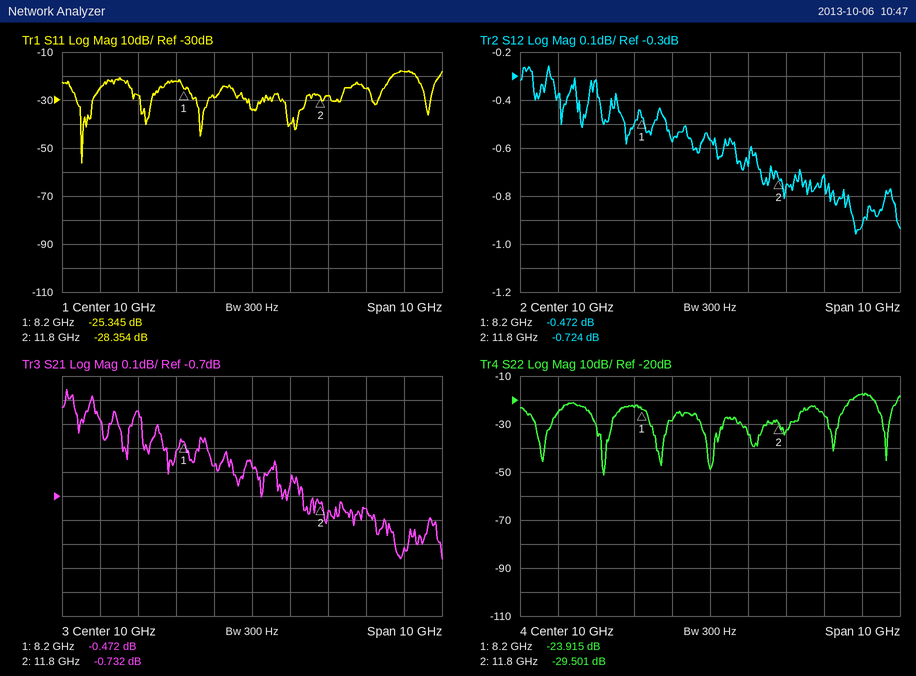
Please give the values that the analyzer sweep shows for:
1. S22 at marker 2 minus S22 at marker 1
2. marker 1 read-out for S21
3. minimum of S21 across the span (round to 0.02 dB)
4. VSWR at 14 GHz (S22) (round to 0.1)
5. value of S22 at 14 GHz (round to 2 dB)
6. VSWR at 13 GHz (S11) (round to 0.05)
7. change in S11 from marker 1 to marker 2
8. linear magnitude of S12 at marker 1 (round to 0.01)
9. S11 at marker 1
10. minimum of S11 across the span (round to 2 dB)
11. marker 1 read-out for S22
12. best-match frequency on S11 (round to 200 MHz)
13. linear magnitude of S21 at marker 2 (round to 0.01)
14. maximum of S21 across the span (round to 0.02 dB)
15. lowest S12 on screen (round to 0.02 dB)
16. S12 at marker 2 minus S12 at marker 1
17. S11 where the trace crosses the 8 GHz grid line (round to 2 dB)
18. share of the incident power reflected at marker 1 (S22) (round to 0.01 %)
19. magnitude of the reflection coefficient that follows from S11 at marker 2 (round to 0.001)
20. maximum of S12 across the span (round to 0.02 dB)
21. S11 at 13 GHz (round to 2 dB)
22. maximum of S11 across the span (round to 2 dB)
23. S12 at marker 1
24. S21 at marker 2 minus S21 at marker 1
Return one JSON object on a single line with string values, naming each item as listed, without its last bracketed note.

{"S22 at marker 2 minus S22 at marker 1": "-5.586 dB", "marker 1 read-out for S21": "-0.472 dB", "minimum of S21 across the span": "-0.96 dB", "VSWR at 14 GHz (S22)": "1.3", "value of S22 at 14 GHz": "-18 dB", "VSWR at 13 GHz (S11)": "1.10", "change in S11 from marker 1 to marker 2": "-3.009 dB", "linear magnitude of S12 at marker 1": "0.95", "S11 at marker 1": "-25.345 dB", "minimum of S11 across the span": "-56 dB", "marker 1 read-out for S22": "-23.915 dB", "best-match frequency on S11": "5.6 GHz", "linear magnitude of S21 at marker 2": "0.92", "maximum of S21 across the span": "-0.26 dB", "lowest S12 on screen": "-0.96 dB", "S12 at marker 2 minus S12 at marker 1": "-0.252 dB", "S11 where the trace crosses the 8 GHz grid line": "-22 dB", "share of the incident power reflected at marker 1 (S22)": "0.41 %", "magnitude of the reflection coefficient that follows from S11 at marker 2": "0.038", "maximum of S12 across the span": "-0.26 dB", "S11 at 13 GHz": "-26 dB", "maximum of S11 across the span": "-18 dB", "S12 at marker 1": "-0.472 dB", "S21 at marker 2 minus S21 at marker 1": "-0.260 dB"}
